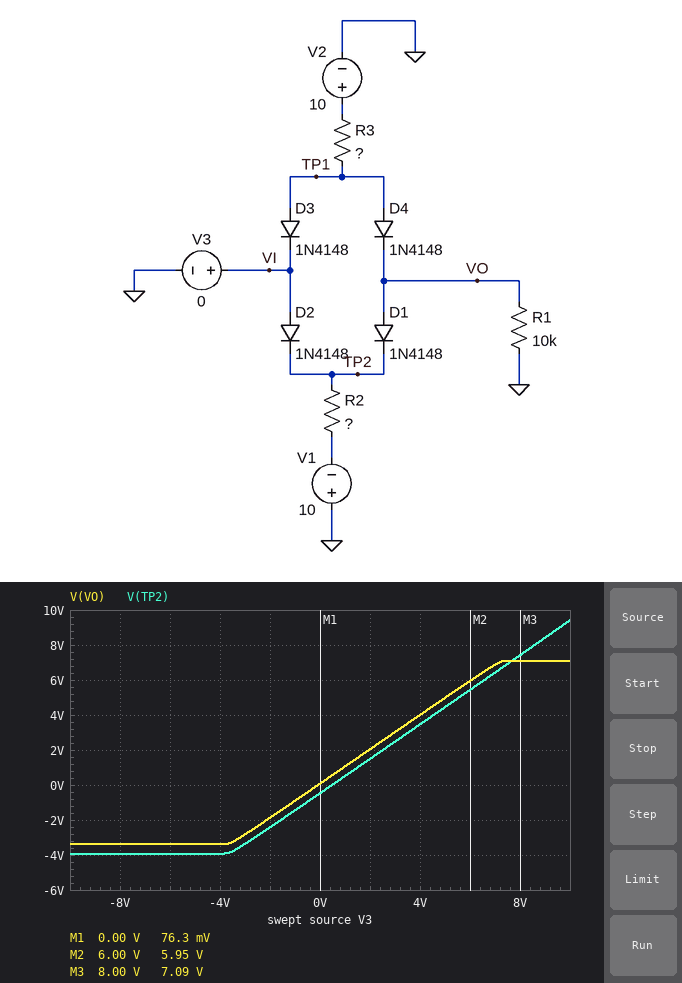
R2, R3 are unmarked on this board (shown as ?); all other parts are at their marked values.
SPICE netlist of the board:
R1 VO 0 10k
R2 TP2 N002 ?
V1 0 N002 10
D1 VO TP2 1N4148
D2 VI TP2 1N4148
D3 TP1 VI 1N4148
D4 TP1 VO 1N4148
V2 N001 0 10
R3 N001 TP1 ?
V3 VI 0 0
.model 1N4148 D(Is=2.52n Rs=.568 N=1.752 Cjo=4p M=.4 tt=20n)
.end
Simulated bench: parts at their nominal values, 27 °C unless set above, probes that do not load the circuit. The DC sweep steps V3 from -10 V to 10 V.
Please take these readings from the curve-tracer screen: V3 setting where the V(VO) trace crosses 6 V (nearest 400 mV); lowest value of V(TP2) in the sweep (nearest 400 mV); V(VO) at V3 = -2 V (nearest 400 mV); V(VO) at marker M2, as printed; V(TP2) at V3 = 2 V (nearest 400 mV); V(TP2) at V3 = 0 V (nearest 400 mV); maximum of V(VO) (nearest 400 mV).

6.0 V
-4.0 V
-2.0 V
5.95 V
1.6 V
-400 mV
7.2 V
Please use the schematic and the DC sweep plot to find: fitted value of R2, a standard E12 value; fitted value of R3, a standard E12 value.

18 kΩ
3.3 kΩ
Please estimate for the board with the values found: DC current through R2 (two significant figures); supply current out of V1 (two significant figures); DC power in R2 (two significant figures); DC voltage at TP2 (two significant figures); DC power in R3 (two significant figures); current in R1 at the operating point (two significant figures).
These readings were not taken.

530 µA
530 µA
5.0 mW
-470 mV
27 mW
7.6 µA
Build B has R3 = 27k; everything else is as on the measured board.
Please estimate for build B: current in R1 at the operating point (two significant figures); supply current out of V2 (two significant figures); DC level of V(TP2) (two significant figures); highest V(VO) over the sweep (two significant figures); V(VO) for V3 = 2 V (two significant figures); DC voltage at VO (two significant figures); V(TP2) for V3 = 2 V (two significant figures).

1.8 µA
350 µA
-530 mV
2.6 V
1.9 V
-18 mV
1.4 V
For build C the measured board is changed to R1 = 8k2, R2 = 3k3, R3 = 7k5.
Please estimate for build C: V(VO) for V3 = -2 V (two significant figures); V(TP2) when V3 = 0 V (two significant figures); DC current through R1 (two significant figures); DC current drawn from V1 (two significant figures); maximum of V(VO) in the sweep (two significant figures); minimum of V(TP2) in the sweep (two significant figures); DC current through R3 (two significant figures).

-2.0 V
-620 mV
4.5 µA
2.8 mA
4.9 V
-7.3 V
1.3 mA
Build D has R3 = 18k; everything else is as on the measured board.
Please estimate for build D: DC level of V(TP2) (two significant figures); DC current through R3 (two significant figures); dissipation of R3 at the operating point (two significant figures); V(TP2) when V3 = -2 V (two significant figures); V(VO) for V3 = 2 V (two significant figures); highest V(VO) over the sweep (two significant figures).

-520 mV
530 µA
5.0 mW
-2.5 V
1.9 V
3.4 V
